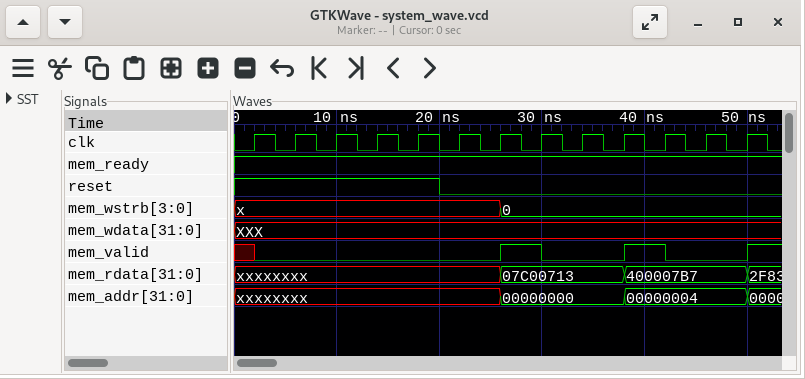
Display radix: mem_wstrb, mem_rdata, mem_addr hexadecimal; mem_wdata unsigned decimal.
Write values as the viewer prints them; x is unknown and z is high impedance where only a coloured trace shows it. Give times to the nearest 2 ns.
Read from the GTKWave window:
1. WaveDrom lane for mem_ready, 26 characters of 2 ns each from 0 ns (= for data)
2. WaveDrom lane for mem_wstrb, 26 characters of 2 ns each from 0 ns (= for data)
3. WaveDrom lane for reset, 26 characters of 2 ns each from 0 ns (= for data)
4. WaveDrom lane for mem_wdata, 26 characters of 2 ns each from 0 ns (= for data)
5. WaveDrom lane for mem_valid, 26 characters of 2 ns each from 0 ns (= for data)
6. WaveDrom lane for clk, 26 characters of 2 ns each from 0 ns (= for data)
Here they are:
{name: 'mem_ready', wave: '1.........................'}
{name: 'mem_wstrb', wave: 'x............=............', data: '0'}
{name: 'reset', wave: '1.........0...............'}
{name: 'mem_wdata', wave: 'x.........................'}
{name: 'mem_valid', wave: 'x0...........1.0...1.0...1'}
{name: 'clk', wave: '01010101010101010101010101'}
